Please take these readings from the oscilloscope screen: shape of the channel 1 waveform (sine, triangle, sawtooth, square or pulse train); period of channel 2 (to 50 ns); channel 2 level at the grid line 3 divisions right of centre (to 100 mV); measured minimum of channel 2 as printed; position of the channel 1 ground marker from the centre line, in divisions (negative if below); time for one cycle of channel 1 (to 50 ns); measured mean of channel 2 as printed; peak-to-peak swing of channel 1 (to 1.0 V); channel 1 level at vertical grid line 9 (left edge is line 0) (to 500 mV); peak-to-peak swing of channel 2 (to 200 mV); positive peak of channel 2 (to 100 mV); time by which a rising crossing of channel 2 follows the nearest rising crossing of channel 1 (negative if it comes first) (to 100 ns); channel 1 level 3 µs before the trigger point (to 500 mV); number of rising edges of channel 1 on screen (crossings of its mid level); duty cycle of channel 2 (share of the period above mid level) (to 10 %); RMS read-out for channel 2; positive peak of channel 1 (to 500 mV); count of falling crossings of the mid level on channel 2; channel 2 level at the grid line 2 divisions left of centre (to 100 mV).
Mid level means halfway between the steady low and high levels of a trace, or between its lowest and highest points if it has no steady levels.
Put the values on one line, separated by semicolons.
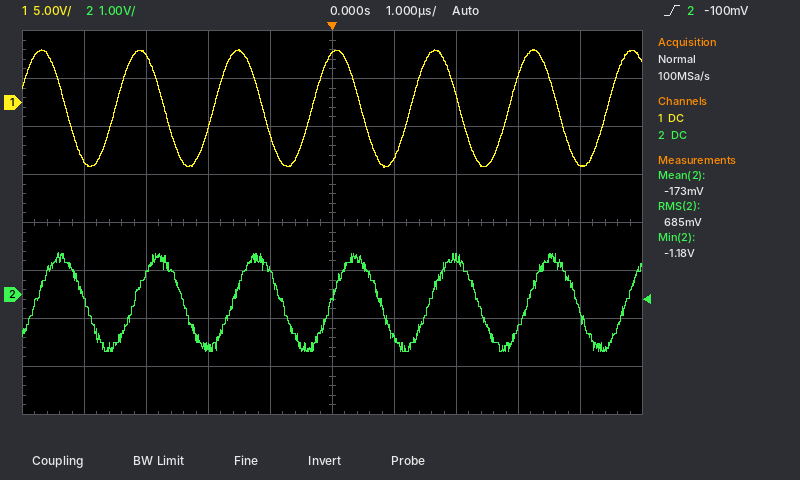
sine; 1.60 µs; -700 mV; -1.18 V; +2.5 div; 1.60 µs; -173 mV; 12.0 V; -6.5 V; 2.0 V; 900 mV; +300 ns; 5.0 V; 6; 50 %; 685 mV; 5.5 V; 6; -1.1 V
